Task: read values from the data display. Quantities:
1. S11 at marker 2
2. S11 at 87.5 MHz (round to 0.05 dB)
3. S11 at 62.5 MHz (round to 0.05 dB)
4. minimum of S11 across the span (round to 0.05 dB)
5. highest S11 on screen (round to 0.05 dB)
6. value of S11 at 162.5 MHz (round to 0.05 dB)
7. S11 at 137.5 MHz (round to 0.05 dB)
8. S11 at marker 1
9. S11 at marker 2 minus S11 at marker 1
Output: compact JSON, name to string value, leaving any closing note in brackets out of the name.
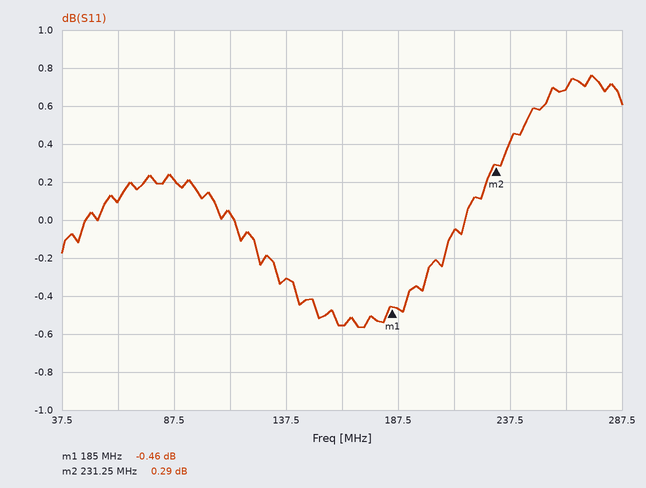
{"S11 at marker 2": "0.29 dB", "S11 at 87.5 MHz": "0.20 dB", "S11 at 62.5 MHz": "0.10 dB", "minimum of S11 across the span": "-0.55 dB", "highest S11 on screen": "0.75 dB", "value of S11 at 162.5 MHz": "-0.55 dB", "S11 at 137.5 MHz": "-0.30 dB", "S11 at marker 1": "-0.46 dB", "S11 at marker 2 minus S11 at marker 1": "0.75 dB"}
